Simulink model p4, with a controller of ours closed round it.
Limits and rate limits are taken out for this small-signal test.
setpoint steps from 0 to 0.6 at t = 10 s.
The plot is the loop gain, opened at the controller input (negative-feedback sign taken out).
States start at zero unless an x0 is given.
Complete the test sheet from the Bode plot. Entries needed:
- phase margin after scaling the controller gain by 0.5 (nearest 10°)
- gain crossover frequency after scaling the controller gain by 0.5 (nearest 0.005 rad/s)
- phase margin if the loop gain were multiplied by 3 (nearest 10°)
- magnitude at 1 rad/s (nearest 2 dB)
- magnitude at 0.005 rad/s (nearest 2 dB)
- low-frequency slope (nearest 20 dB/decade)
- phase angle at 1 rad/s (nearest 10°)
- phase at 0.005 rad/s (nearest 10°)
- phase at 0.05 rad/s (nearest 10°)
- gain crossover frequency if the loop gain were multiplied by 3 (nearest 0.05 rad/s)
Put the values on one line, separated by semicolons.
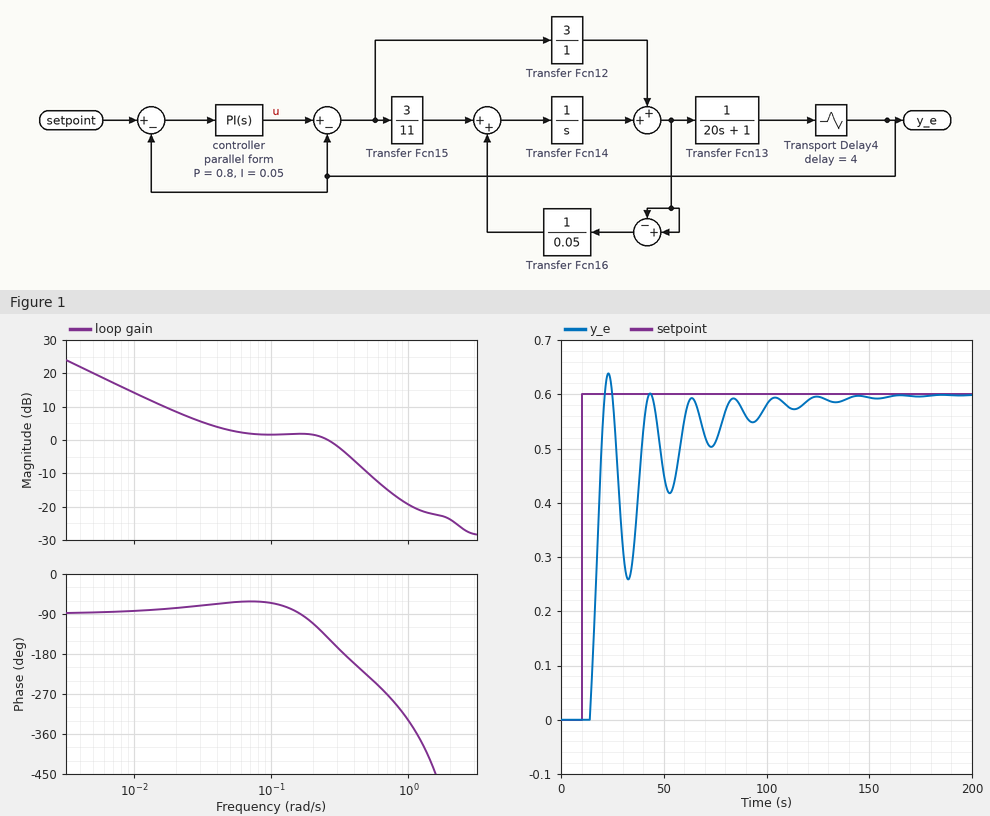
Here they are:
110°; 0.030 rad/s; -50°; -20 dB; 20 dB; -20 dB/decade; -330°; -90°; -60°; 0.50 rad/s
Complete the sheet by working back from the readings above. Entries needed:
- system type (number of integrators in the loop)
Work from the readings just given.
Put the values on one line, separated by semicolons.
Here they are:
1
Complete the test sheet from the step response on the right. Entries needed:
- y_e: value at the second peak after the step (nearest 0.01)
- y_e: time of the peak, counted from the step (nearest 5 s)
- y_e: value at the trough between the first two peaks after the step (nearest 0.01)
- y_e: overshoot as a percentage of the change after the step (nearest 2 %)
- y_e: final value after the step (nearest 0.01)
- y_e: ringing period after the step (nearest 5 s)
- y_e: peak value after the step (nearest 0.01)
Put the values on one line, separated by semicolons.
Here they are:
0.60; 15 s; 0.26; 6 %; 0.60; 20 s; 0.64
